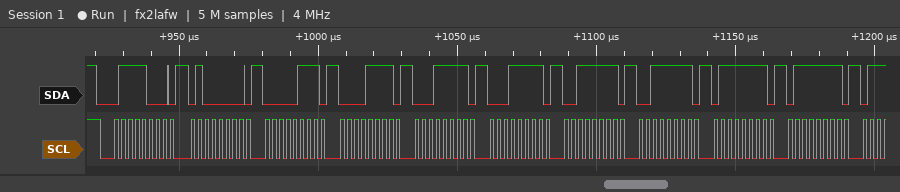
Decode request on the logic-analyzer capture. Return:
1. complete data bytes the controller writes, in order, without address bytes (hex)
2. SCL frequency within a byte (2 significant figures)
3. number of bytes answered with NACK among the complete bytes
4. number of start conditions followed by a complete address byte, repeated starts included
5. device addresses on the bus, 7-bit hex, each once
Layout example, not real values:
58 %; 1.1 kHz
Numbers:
40 07 0F 1F 1F 3F 3F 7F 7F; 400 kHz; 0; 1; 0x3C
